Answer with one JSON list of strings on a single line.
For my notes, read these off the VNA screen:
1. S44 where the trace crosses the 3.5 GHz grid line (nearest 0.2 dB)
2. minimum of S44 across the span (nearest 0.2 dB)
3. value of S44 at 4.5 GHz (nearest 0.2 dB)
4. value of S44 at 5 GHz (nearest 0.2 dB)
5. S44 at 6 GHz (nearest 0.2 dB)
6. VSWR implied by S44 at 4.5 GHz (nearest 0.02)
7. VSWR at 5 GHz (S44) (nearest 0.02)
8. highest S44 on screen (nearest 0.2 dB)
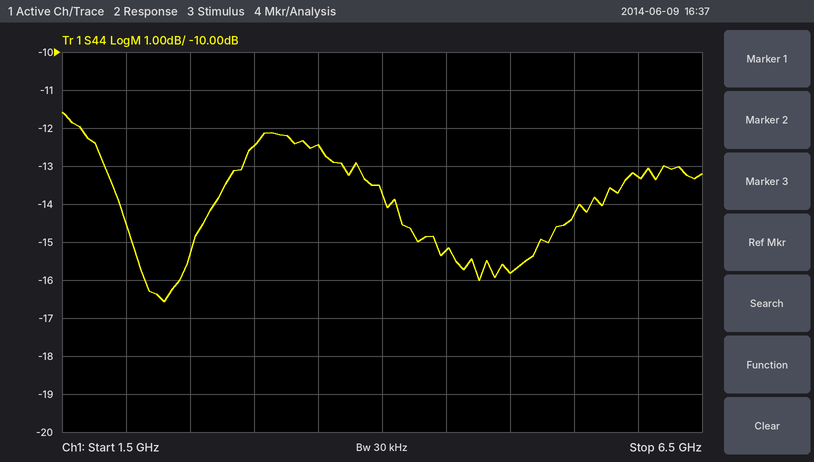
["-12.4 dB", "-16.6 dB", "-15.2 dB", "-15.8 dB", "-13.2 dB", "1.42", "1.38", "-11.6 dB"]
